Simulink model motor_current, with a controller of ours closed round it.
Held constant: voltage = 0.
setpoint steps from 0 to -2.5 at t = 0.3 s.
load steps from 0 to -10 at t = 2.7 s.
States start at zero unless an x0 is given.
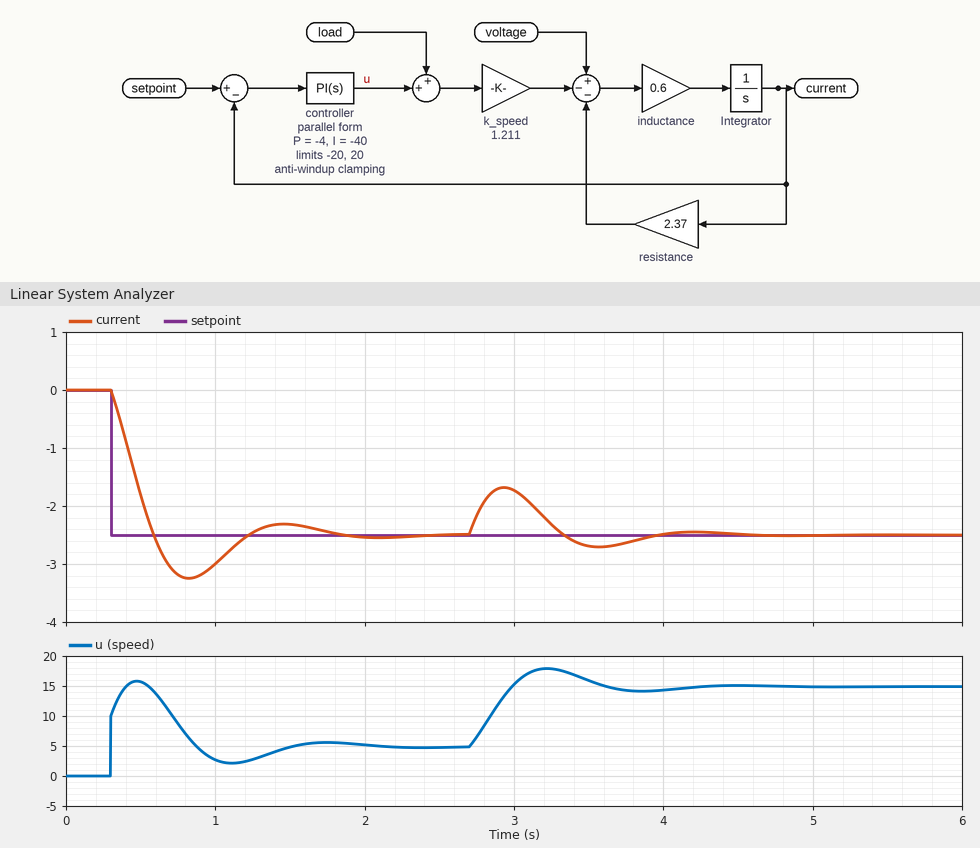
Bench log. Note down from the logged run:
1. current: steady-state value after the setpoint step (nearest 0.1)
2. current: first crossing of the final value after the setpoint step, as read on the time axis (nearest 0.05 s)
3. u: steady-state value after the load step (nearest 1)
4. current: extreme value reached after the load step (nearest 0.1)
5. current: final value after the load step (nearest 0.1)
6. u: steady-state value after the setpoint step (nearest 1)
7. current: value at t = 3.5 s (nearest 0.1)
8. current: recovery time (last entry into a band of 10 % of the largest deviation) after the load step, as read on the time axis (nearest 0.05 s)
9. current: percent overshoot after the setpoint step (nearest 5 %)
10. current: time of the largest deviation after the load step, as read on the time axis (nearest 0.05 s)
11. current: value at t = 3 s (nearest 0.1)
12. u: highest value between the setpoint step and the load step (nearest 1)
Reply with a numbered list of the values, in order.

1. -2.5
2. 0.60 s
3. 15
4. -1.7
5. -2.5
6. 5
7. -2.7
8. 3.85 s
9. 30 %
10. 2.95 s
11. -1.7
12. 16
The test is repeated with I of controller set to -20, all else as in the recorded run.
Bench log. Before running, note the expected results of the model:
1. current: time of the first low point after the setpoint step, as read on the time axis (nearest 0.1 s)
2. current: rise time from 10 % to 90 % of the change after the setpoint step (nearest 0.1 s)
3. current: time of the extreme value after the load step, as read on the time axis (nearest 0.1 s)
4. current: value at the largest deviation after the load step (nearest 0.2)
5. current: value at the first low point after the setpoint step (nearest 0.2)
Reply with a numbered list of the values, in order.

1. 1.0 s
2. 0.3 s
3. 3.0 s
4. -1.6
5. -3.0
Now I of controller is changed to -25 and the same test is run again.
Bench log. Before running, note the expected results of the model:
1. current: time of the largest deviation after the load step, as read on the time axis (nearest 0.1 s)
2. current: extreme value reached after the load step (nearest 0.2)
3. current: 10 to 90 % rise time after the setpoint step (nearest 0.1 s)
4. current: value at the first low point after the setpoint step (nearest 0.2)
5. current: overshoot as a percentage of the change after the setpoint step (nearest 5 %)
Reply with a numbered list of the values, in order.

1. 3.0 s
2. -1.6
3. 0.3 s
4. -3.0
5. 20 %
